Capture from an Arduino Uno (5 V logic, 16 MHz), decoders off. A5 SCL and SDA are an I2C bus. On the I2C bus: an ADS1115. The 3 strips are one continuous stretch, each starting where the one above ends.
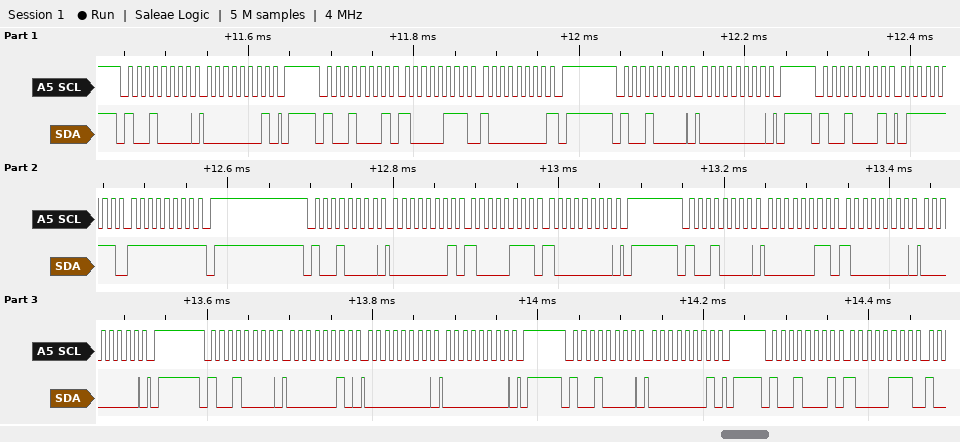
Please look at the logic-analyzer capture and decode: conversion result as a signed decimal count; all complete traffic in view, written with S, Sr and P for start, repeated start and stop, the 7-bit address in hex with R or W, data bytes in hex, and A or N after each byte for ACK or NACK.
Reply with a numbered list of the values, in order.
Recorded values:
1. 32767
2. S 48W A 01 A P S 48R A 87 A 80 N P S 48W A 00 A P S 48R A 7F A FF N P S 48W A 01 A 87 A 80 A P S 48W A 03 A 80 A 00 A P S 48W A 02 A 00 A 00 A P S 48W A 01 A P S 48R A 87 A
